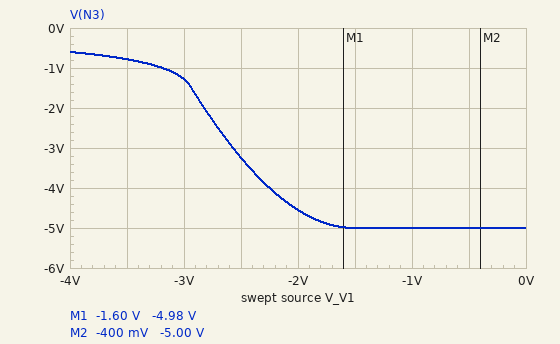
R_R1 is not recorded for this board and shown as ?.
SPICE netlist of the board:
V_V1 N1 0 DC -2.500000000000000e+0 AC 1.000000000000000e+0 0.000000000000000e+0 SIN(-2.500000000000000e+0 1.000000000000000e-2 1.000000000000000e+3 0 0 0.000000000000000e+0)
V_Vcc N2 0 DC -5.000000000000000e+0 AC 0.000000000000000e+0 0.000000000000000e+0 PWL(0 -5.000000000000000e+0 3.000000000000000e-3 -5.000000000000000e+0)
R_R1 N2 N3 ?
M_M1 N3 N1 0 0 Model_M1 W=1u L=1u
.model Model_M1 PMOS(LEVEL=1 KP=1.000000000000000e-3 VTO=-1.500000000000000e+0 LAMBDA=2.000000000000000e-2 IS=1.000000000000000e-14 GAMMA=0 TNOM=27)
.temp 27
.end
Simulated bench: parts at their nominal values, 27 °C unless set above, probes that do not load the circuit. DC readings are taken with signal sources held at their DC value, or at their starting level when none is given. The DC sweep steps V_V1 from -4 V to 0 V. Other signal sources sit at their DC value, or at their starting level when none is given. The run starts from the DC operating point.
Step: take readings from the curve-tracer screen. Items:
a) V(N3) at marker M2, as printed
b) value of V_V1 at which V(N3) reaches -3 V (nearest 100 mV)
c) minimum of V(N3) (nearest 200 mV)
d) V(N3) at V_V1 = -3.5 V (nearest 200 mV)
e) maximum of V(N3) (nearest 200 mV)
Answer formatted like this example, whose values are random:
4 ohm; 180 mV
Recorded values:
-5.00 V; -2.6 V; -5.0 V; -800 mV; -600 mV
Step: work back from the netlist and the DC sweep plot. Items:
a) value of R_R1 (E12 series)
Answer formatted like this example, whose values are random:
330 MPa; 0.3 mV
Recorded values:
3.3 kΩ
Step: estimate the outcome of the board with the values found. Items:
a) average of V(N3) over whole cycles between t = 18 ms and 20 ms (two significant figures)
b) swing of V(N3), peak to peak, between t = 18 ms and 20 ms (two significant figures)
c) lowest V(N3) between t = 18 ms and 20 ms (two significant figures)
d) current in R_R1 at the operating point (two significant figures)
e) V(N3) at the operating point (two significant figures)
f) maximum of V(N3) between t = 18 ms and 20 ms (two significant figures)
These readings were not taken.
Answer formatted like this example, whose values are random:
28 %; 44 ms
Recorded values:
-3.2 V; 68 mV; -3.3 V; 530 µA; -3.2 V; -3.2 V
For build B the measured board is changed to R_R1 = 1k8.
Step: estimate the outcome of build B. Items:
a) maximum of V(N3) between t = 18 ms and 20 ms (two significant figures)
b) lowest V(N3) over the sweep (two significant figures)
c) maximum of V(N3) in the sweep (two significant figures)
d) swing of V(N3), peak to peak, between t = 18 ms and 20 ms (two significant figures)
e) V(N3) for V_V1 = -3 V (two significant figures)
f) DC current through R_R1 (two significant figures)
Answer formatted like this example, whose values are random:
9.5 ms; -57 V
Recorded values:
-4.0 V; -5.0 V; -1.1 V; 38 mV; -2.9 V; 540 µA
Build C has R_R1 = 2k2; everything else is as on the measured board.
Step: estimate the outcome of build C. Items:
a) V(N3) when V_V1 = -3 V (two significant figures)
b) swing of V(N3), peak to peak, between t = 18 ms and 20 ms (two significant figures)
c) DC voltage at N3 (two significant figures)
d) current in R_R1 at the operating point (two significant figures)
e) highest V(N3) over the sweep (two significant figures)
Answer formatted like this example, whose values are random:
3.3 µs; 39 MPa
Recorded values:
-2.4 V; 46 mV; -3.8 V; 540 µA; -890 mV
